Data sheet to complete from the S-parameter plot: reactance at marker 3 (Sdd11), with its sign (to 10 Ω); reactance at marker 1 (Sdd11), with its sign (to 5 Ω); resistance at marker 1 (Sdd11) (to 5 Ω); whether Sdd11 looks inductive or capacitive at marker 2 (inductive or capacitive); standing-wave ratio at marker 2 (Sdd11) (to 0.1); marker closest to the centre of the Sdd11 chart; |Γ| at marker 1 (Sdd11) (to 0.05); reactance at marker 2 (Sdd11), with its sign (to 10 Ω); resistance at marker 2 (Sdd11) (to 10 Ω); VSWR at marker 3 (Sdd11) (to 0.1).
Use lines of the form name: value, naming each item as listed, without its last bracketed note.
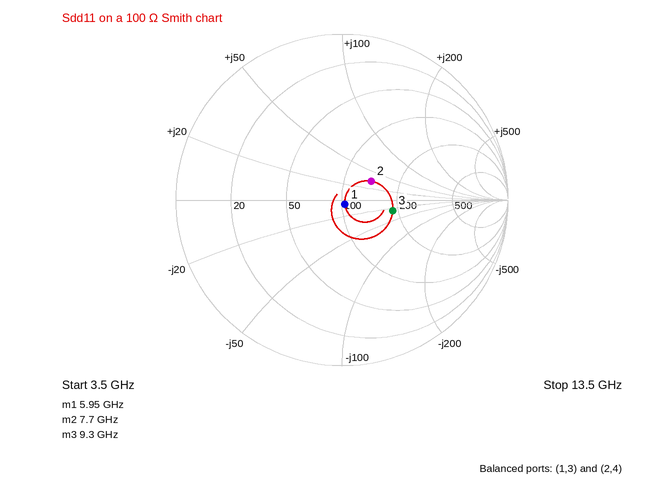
reactance at marker 3 (Sdd11), with its sign: -30 Ω
reactance at marker 1 (Sdd11), with its sign: -5 Ω
resistance at marker 1 (Sdd11): 105 Ω
whether Sdd11 looks inductive or capacitive at marker 2: inductive
standing-wave ratio at marker 2 (Sdd11): 1.5
marker closest to the centre of the Sdd11 chart: marker 1
|Γ| at marker 1 (Sdd11): 0.05
reactance at marker 2 (Sdd11), with its sign: +30 Ω
resistance at marker 2 (Sdd11): 140 Ω
VSWR at marker 3 (Sdd11): 1.9
